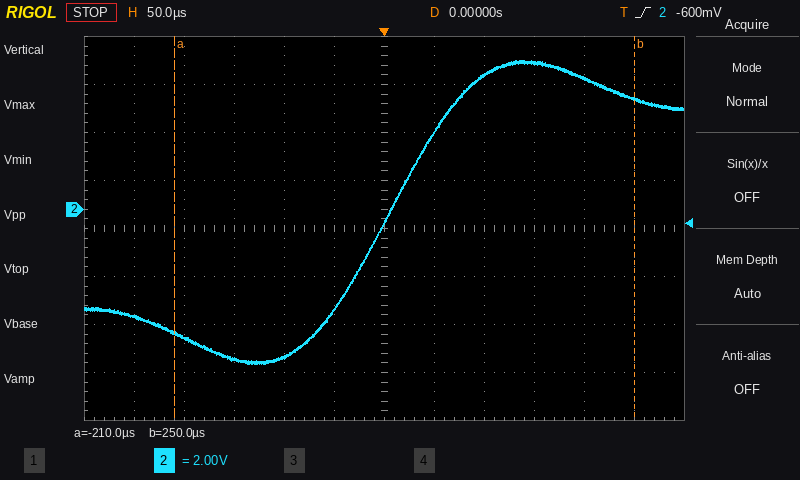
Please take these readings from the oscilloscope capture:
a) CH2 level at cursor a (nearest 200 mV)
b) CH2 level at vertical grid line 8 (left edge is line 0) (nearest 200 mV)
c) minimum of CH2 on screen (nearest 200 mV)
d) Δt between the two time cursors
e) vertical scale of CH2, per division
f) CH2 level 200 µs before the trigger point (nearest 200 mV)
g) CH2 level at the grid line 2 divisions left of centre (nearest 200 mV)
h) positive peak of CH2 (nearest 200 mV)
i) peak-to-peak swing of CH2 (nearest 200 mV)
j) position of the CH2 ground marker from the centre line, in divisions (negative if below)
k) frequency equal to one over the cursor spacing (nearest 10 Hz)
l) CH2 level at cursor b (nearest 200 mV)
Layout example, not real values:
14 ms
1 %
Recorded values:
-5.2 V
5.6 V
-6.4 V
460 µs
2 V
-5.4 V
-6.2 V
6.2 V
12.6 V
+0.4 div
2.17 kHz
4.6 V
